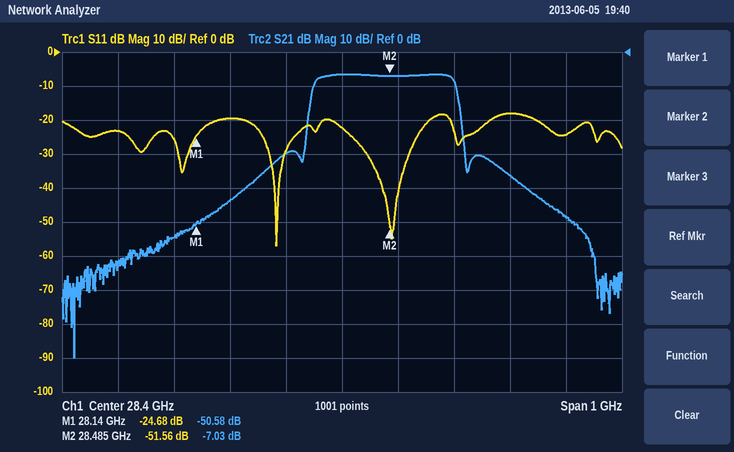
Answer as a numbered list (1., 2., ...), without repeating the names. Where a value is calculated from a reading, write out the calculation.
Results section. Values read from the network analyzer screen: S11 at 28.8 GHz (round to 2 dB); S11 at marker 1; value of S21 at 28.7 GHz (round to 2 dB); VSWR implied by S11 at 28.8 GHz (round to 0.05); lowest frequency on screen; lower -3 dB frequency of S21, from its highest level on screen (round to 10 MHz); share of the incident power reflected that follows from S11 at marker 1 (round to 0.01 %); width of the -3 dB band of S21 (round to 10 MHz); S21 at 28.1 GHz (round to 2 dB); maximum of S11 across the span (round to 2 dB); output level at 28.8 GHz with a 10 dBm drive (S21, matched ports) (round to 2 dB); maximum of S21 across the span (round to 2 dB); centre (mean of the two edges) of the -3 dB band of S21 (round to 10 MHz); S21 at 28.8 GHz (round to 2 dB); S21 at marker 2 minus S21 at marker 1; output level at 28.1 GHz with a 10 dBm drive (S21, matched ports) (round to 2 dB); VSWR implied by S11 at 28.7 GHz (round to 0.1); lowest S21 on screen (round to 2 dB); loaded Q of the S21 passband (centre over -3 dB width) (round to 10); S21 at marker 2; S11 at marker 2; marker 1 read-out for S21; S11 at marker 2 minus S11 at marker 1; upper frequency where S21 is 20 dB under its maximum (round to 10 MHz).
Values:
1. -24 dB
2. -24.68 dB
3. -36 dB
4. |Γ| = 10^(-24/20) = 0.0631; VSWR = (1 + 0.0631)/(1 − 0.0631) ≈ 1.13, so 1.15 to the nearest 0.05
5. 27.9 GHz
6. 28.35 GHz
7. 10^(-24.68/10) ≈ 0.34 %
8. 28.60 GHz − 28.35 GHz = 250 MHz
9. -54 dB
10. -18 dB
11. 10 dBm + (-48 dB) = -38 dBm
12. -6 dB
13. 28.48 GHz
14. -48 dB
15. -7.03 − (-50.58) = 43.55 dB
16. 10 dBm + (-54 dB) = -44 dBm
17. |Γ| = 10^(-18/20) = 0.1259; VSWR = (1 + 0.1259)/(1 − 0.1259) ≈ 1.3
18. -90 dB
19. 28.475 GHz / 250 MHz ≈ 114, so 110 to the nearest 10
20. -7.03 dB
21. -51.56 dB
22. -50.58 dB
23. -51.56 − (-24.68) = -26.88 dB
24. 28.62 GHz
